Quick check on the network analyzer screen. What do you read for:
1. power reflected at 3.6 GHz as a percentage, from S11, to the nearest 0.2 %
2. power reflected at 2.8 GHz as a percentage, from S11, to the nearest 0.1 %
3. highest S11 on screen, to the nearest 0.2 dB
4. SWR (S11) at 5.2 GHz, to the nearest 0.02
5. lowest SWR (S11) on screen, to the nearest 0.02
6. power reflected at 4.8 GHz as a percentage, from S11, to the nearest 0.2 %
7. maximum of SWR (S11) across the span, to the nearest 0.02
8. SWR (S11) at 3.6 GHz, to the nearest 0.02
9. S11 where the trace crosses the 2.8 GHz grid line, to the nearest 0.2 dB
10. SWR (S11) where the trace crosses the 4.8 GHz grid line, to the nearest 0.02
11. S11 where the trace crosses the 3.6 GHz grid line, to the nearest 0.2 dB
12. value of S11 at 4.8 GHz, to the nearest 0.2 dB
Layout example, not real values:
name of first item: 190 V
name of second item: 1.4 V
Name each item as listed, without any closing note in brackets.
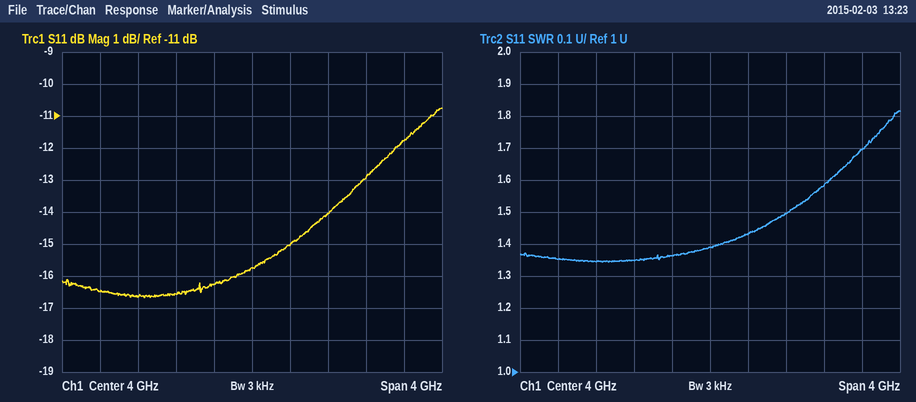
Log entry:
power reflected at 3.6 GHz as a percentage, from S11, to the nearest 0.2 %: 2.4 %
power reflected at 2.8 GHz as a percentage, from S11, to the nearest 0.1 %: 2.2 %
highest S11 on screen, to the nearest 0.2 dB: -10.8 dB
SWR (S11) at 5.2 GHz, to the nearest 0.02: 1.58
lowest SWR (S11) on screen, to the nearest 0.02: 1.34
power reflected at 4.8 GHz as a percentage, from S11, to the nearest 0.2 %: 4.0 %
maximum of SWR (S11) across the span, to the nearest 0.02: 1.82
SWR (S11) at 3.6 GHz, to the nearest 0.02: 1.36
S11 where the trace crosses the 2.8 GHz grid line, to the nearest 0.2 dB: -16.6 dB
SWR (S11) where the trace crosses the 4.8 GHz grid line, to the nearest 0.02: 1.50
S11 where the trace crosses the 3.6 GHz grid line, to the nearest 0.2 dB: -16.2 dB
value of S11 at 4.8 GHz, to the nearest 0.2 dB: -14.0 dB
